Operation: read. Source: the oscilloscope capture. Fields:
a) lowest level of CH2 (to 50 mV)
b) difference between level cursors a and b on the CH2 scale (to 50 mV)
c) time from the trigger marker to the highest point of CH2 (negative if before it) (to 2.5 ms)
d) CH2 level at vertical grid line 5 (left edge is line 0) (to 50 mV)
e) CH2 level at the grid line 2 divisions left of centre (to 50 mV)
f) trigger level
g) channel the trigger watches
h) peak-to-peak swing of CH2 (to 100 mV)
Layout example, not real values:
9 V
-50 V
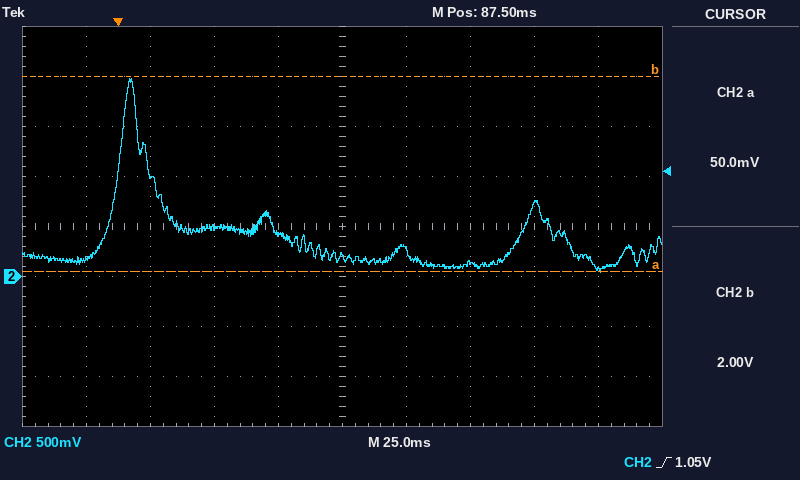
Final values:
50 mV
1.95 V
+5.0 ms
200 mV
500 mV
1.05 V
CH2
1.90 V
